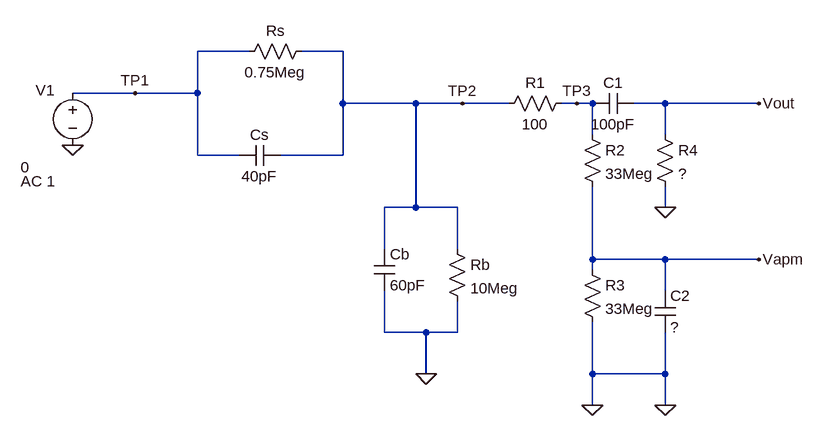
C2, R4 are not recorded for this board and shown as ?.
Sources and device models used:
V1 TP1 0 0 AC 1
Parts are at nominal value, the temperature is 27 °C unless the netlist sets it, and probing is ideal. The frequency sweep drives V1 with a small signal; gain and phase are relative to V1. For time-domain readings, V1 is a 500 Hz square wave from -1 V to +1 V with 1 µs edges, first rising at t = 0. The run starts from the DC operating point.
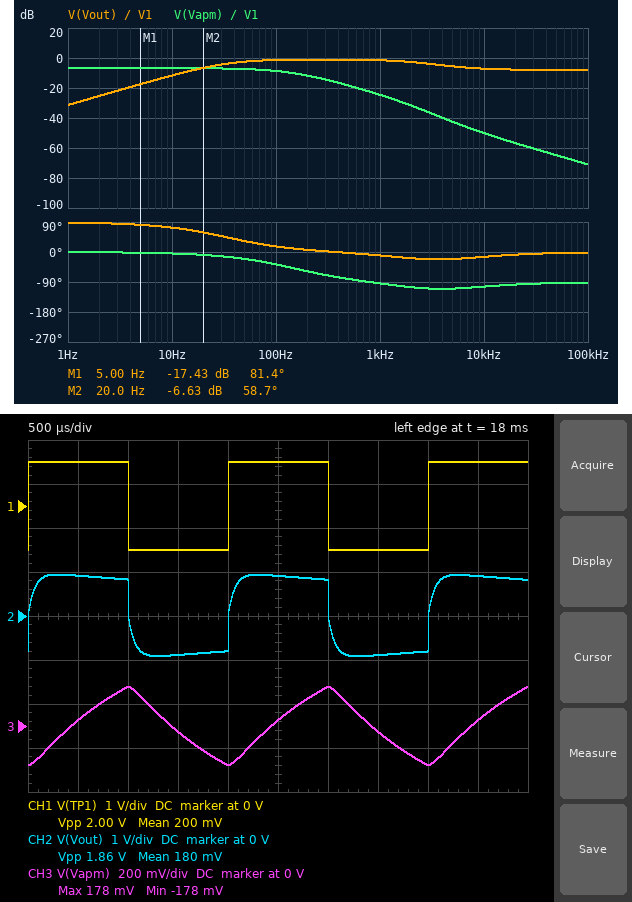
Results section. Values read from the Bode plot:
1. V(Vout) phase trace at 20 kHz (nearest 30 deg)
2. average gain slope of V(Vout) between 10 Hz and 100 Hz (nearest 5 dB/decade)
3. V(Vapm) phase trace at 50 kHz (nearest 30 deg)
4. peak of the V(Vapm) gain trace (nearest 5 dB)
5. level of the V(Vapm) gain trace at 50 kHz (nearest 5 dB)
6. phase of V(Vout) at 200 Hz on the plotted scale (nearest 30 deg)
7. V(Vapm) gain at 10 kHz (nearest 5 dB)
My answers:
0 deg
10 dB/decade
-90 deg
-5 dB
-65 dB
0 deg
-50 dB
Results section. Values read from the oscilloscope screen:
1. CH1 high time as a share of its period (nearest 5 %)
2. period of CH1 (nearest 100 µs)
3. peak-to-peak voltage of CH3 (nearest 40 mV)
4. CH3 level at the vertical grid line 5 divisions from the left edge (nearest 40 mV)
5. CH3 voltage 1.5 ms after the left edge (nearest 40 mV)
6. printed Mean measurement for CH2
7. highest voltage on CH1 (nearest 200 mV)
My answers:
50 %
2.0 ms
360 mV
40 mV
-40 mV
180 mV
1.0 V
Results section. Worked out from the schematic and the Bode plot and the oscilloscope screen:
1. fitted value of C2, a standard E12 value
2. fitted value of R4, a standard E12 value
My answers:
68 pF
47 MΩ
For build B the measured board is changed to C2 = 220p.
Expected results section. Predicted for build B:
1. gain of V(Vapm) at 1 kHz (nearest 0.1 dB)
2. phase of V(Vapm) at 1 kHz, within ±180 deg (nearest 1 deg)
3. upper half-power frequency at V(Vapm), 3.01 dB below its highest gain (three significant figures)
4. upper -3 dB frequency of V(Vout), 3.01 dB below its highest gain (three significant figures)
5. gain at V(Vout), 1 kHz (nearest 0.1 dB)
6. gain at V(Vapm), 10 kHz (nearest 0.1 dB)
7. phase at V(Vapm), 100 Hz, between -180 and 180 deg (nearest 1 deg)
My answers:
-34.7 dB
-100 deg
42.6 Hz
3.15 kHz
-1.5 dB
-60.3 dB
-68 deg
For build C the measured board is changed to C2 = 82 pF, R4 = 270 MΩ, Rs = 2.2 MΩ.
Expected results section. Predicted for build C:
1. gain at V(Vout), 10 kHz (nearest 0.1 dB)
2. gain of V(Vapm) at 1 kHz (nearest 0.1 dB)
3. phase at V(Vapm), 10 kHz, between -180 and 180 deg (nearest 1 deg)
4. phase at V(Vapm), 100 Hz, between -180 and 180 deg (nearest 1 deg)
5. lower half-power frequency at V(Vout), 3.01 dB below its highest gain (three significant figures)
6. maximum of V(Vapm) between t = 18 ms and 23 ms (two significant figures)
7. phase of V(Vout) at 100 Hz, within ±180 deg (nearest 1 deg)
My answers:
-7.9 dB
-29.1 dB
-94 deg
-44 deg
5.72 Hz
120 mV
0 deg
